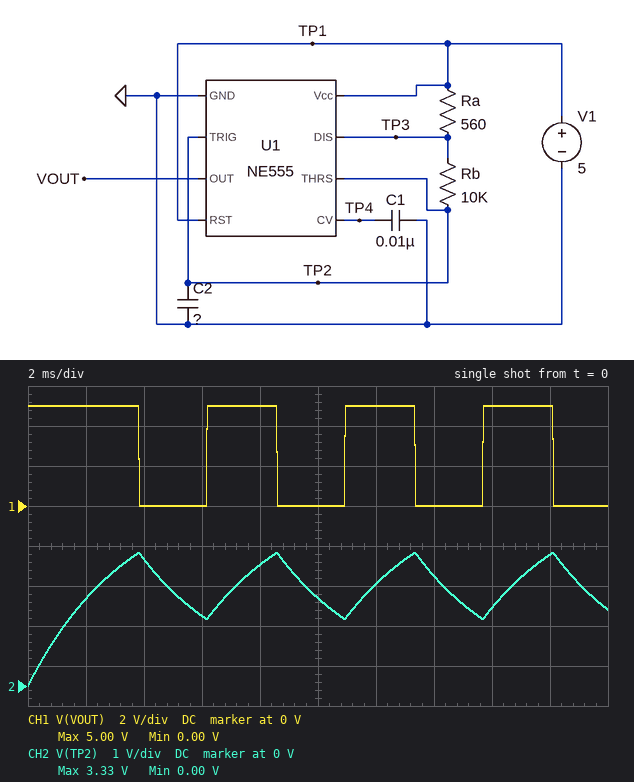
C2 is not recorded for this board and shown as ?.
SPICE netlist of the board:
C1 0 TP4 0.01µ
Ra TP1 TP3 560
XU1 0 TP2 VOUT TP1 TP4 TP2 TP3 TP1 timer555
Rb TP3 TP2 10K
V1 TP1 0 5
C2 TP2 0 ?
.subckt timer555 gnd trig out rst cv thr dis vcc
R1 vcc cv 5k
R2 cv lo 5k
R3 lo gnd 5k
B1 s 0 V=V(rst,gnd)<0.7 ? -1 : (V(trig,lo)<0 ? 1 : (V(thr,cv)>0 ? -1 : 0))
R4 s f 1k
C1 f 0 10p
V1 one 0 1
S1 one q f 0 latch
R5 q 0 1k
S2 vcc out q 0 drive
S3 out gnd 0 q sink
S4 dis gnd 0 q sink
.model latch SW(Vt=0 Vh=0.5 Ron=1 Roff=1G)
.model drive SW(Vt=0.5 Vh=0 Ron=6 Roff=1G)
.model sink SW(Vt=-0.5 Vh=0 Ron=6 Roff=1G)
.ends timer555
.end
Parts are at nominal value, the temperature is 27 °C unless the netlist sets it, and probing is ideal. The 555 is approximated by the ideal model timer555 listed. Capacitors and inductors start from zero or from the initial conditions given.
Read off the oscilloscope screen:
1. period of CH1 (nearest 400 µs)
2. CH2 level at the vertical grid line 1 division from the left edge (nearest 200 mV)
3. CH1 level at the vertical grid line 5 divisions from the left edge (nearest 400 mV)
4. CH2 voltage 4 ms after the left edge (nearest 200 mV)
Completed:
4.8 ms
2.2 V
0 V
3.2 V
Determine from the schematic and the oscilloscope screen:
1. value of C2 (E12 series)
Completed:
330 nF
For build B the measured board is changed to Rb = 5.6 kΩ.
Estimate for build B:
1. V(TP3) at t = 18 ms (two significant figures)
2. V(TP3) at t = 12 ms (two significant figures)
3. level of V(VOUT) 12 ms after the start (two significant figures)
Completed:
4.8 V
4.7 V
5.0 V
